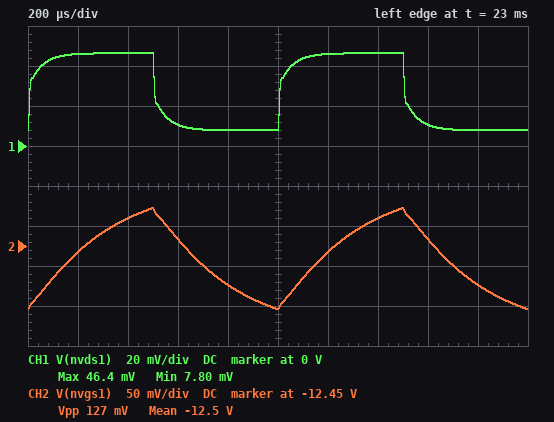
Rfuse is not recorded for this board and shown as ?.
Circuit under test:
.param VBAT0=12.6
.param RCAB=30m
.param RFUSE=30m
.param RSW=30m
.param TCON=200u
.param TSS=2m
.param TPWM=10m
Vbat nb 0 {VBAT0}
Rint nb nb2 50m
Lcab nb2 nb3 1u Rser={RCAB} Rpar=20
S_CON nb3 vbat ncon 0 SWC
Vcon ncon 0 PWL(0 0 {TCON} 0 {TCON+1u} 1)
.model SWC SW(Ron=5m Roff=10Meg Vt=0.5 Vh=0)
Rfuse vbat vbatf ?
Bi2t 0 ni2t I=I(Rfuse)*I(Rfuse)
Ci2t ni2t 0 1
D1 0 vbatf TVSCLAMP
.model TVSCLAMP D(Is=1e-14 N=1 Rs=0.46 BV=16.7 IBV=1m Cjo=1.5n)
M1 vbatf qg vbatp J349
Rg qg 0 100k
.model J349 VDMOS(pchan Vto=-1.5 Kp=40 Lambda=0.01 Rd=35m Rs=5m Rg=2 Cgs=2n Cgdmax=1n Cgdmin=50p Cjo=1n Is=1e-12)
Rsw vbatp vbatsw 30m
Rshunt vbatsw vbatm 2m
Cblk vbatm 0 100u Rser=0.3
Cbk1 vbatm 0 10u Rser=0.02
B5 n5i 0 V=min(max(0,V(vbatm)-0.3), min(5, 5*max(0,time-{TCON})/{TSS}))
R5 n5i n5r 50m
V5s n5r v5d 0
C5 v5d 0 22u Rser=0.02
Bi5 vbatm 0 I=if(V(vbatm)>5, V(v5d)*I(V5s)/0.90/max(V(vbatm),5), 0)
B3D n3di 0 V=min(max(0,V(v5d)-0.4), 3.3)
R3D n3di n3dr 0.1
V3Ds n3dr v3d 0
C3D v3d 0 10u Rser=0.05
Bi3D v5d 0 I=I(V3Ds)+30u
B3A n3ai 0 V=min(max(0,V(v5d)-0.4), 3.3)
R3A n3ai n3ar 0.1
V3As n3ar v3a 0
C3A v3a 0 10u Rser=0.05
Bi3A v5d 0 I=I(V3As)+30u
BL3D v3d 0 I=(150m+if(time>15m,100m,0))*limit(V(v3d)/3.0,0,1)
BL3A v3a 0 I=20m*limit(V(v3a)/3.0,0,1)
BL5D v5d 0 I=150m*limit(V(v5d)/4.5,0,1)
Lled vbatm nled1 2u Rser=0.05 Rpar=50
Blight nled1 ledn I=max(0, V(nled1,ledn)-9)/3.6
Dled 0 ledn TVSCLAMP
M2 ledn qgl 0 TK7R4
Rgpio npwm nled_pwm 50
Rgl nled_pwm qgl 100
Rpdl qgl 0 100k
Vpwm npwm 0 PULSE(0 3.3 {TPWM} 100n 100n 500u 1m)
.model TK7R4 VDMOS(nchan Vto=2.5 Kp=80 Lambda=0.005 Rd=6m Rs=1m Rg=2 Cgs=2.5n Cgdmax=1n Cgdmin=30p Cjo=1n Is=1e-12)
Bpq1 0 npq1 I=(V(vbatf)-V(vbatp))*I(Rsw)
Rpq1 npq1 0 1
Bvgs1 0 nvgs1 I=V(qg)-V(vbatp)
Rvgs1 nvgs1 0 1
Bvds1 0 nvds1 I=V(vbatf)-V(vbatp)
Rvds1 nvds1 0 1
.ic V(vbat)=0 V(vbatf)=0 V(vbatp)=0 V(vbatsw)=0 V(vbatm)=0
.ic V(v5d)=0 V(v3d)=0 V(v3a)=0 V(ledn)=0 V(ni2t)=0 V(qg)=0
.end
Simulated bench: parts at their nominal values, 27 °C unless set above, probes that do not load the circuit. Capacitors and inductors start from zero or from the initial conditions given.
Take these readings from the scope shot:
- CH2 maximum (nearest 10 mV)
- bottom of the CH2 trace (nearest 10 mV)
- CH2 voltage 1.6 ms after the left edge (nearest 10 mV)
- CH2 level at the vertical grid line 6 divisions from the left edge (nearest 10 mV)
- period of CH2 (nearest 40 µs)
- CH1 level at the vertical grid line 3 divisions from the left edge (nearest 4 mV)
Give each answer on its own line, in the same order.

-12.40 V
-12.53 V
-12.44 V
-12.46 V
1.00 ms
12 mV
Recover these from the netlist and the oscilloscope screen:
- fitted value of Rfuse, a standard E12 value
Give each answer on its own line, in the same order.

0.082 Ω
